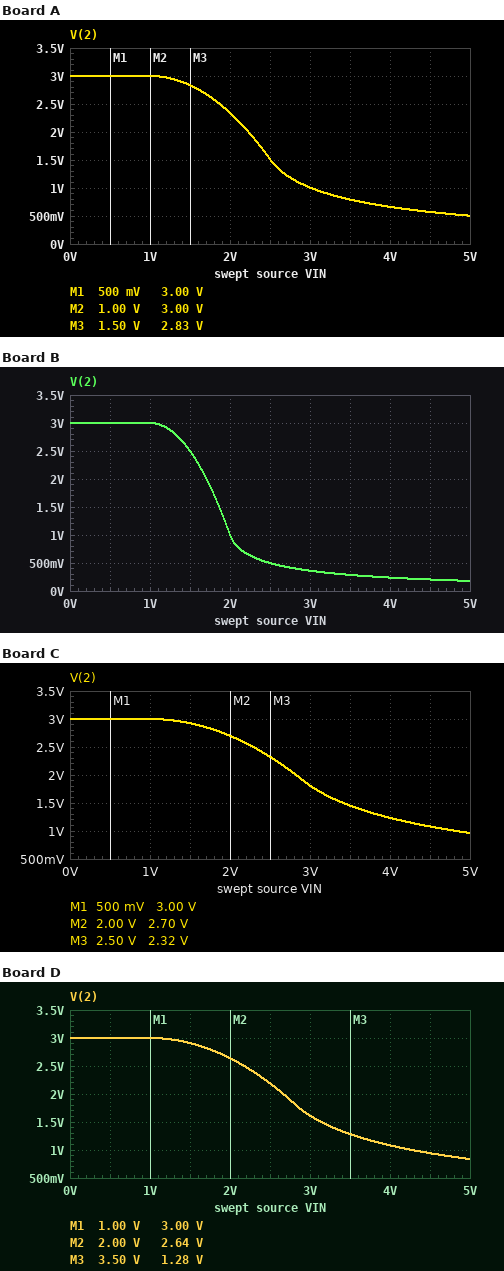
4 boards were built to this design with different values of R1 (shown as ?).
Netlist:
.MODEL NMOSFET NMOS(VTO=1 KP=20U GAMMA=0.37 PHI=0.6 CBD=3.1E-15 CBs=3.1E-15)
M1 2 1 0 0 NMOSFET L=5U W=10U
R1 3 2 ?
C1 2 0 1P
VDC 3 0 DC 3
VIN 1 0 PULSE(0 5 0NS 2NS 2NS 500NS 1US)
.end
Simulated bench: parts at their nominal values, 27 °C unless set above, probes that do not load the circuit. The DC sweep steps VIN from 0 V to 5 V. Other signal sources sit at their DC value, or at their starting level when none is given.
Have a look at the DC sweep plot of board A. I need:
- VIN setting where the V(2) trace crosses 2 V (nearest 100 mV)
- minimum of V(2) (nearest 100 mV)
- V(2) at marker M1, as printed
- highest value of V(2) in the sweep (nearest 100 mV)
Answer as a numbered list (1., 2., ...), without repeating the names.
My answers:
1. 2.2 V
2. 500 mV
3. 3.00 V
4. 3.0 V
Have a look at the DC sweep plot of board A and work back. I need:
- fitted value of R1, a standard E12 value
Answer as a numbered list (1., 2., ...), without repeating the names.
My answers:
1. 33 kΩ
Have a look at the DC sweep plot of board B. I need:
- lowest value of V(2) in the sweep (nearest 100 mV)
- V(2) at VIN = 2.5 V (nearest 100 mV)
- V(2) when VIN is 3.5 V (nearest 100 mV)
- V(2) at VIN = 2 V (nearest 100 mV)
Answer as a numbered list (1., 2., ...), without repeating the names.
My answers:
1. 200 mV
2. 500 mV
3. 300 mV
4. 1.0 V
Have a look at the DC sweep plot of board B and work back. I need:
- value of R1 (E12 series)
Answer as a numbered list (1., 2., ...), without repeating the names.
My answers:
1. 100 kΩ
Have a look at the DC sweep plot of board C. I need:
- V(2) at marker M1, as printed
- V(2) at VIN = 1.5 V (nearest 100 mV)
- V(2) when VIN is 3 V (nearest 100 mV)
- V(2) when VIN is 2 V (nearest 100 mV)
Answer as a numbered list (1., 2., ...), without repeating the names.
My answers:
1. 3.00 V
2. 2.9 V
3. 1.8 V
4. 2.7 V
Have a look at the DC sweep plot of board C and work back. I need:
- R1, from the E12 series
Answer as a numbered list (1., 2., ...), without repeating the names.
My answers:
1. 15 kΩ
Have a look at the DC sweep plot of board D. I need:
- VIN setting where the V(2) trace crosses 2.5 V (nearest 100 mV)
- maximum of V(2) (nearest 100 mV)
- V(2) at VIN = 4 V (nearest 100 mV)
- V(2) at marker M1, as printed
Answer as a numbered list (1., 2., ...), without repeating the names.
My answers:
1. 2.2 V
2. 3.0 V
3. 1.1 V
4. 3.00 V
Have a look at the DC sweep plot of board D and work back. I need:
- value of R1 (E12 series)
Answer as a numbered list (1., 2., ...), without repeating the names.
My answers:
1. 18 kΩ
